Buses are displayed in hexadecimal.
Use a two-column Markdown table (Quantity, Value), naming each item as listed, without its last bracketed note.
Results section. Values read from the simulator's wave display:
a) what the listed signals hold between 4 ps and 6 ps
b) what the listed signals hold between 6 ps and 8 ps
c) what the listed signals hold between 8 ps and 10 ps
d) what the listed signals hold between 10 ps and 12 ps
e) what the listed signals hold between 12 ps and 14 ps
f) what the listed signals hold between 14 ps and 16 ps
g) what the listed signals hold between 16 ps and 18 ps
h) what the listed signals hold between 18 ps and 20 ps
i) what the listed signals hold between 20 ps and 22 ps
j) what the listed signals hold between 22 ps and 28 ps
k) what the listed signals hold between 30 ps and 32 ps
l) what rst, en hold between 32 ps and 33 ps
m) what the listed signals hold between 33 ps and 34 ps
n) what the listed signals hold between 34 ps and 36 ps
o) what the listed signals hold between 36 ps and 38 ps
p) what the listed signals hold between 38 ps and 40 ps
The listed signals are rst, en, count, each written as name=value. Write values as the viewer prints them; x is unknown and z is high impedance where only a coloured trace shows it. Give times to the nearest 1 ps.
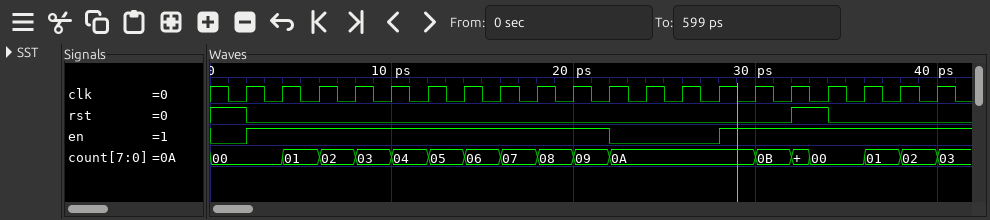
| Quantity | Value |
|---|---|
| what the listed signals hold between 4 ps and 6 ps | rst=0, en=1, count=01 |
| what the listed signals hold between 6 ps and 8 ps | rst=0, en=1, count=02 |
| what the listed signals hold between 8 ps and 10 ps | rst=0, en=1, count=03 |
| what the listed signals hold between 10 ps and 12 ps | rst=0, en=1, count=04 |
| what the listed signals hold between 12 ps and 14 ps | rst=0, en=1, count=05 |
| what the listed signals hold between 14 ps and 16 ps | rst=0, en=1, count=06 |
| what the listed signals hold between 16 ps and 18 ps | rst=0, en=1, count=07 |
| what the listed signals hold between 18 ps and 20 ps | rst=0, en=1, count=08 |
| what the listed signals hold between 20 ps and 22 ps | rst=0, en=1, count=09 |
| what the listed signals hold between 22 ps and 28 ps | rst=0, en=0, count=0A |
| what the listed signals hold between 30 ps and 32 ps | rst=0, en=1, count=0B |
| what rst, en hold between 32 ps and 33 ps | rst=1, en=1 |
| what the listed signals hold between 33 ps and 34 ps | rst=1, en=1, count=00 |
| what the listed signals hold between 34 ps and 36 ps | rst=0, en=1, count=00 |
| what the listed signals hold between 36 ps and 38 ps | rst=0, en=1, count=01 |
| what the listed signals hold between 38 ps and 40 ps | rst=0, en=1, count=02 |
